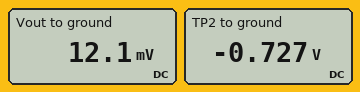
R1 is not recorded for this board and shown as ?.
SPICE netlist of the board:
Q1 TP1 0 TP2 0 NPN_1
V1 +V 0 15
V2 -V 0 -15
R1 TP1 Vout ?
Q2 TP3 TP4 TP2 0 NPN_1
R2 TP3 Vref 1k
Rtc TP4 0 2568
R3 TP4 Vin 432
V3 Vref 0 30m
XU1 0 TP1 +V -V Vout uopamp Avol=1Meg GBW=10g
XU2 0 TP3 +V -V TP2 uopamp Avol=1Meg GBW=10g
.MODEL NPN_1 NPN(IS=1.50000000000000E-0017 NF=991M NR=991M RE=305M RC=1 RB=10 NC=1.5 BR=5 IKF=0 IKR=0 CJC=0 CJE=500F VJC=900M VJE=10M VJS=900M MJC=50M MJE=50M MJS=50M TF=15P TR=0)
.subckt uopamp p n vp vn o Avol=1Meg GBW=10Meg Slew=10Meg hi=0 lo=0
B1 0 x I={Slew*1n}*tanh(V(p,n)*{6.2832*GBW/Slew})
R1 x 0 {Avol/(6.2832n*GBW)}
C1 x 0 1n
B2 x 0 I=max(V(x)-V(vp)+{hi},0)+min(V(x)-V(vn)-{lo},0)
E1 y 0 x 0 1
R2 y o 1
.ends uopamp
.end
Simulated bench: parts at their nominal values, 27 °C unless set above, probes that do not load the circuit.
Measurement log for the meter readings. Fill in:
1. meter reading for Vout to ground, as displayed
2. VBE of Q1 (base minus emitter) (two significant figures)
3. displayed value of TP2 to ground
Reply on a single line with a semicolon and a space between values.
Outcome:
12.1 mV; 730 mV; -0.727 V
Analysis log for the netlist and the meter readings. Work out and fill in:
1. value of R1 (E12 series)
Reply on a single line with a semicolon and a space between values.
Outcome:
390 Ω
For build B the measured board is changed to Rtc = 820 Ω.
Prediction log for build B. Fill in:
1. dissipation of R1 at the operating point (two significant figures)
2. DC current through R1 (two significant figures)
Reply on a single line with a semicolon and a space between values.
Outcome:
360 nW; 30 µA
